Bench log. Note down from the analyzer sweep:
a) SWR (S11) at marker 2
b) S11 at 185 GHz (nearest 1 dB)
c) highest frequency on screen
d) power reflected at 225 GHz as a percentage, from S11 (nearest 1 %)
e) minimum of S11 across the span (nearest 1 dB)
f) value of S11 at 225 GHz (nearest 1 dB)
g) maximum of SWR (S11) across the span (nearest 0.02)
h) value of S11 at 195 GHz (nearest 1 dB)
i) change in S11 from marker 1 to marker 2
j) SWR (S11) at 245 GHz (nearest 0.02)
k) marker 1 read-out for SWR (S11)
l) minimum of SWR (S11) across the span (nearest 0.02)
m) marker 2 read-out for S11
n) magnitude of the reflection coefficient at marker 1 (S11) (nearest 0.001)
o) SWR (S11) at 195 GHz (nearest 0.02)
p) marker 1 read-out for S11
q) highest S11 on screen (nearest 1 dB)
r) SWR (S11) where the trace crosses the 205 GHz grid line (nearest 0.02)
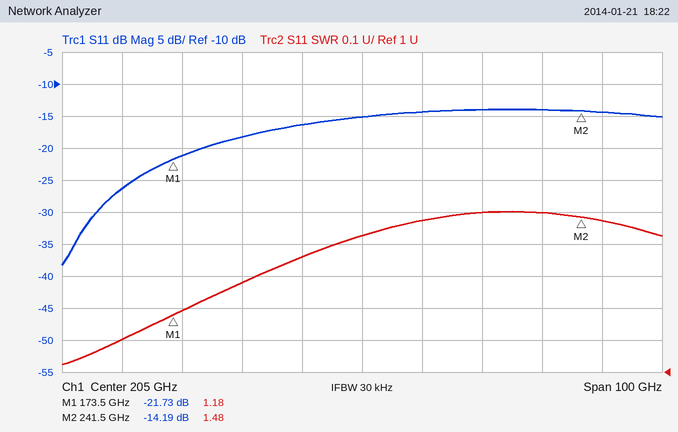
1.48
-18 dB
255 GHz
4 %
-38 dB
-14 dB
1.50
-16 dB
7.54 dB
1.48
1.18
1.02
-14.19 dB
0.082
1.36
-21.73 dB
-14 dB
1.42
